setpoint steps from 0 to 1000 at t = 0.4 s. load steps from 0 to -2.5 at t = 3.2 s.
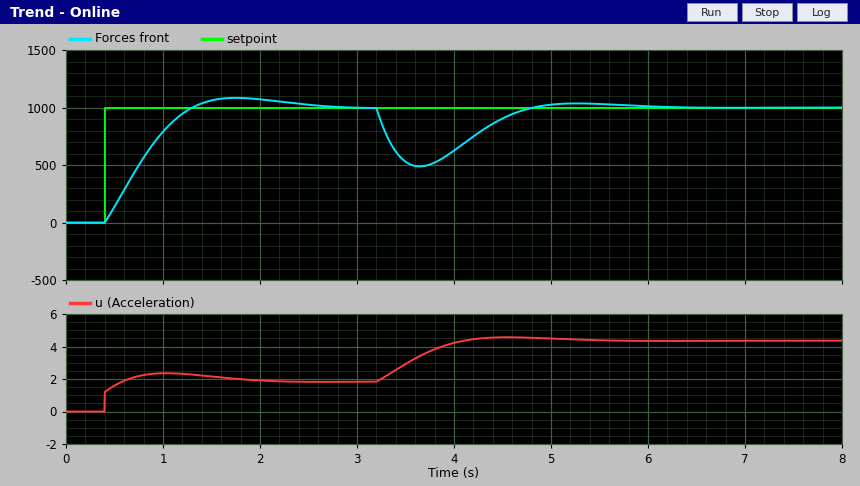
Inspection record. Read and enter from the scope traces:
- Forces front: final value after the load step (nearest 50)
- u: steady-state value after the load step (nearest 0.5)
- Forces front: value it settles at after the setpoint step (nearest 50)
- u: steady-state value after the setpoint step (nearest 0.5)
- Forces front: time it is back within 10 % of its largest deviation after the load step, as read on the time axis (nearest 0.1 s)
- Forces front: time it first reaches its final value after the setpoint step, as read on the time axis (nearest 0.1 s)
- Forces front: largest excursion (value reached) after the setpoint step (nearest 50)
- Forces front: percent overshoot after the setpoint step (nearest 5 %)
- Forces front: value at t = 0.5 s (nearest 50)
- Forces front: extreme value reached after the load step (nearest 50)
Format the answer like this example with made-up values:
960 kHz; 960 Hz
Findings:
1000; 4.5; 1000; 2.0; 4.6 s; 1.3 s; 1100; 10 %; 150; 500
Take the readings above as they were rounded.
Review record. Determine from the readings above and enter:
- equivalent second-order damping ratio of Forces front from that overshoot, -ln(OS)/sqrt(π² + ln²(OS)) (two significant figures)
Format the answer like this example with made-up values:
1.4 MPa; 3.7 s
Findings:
0.59
